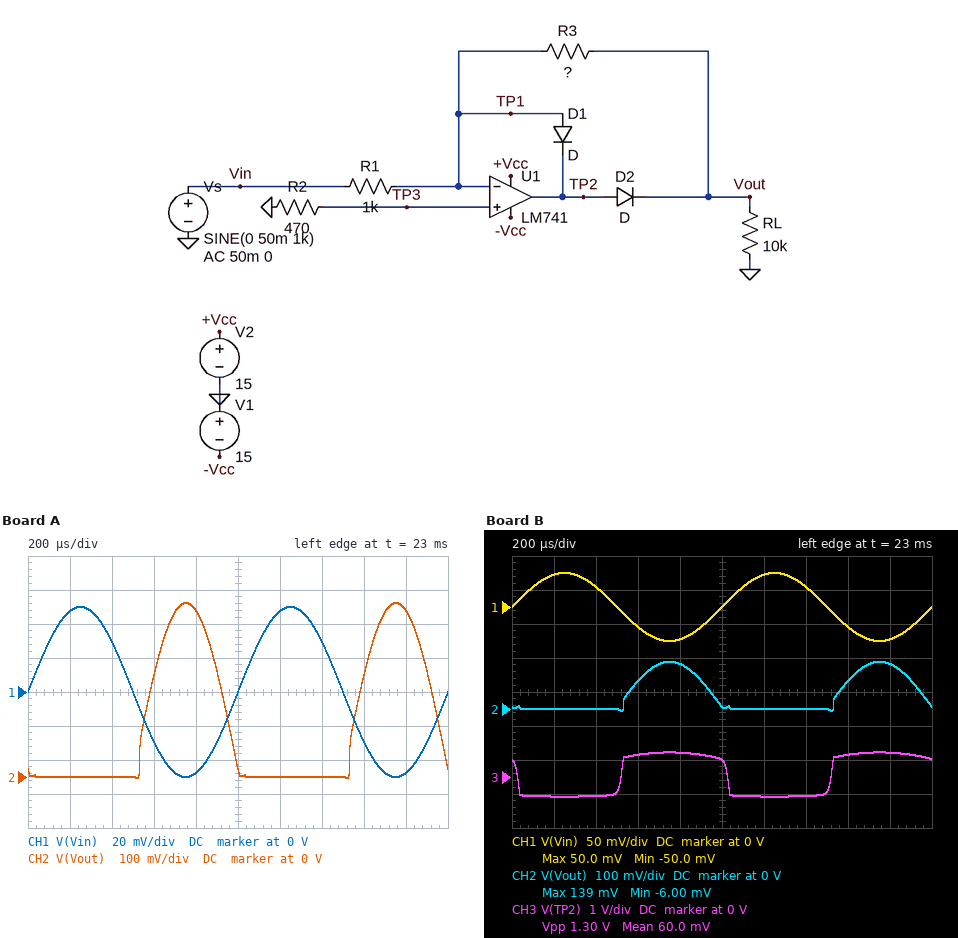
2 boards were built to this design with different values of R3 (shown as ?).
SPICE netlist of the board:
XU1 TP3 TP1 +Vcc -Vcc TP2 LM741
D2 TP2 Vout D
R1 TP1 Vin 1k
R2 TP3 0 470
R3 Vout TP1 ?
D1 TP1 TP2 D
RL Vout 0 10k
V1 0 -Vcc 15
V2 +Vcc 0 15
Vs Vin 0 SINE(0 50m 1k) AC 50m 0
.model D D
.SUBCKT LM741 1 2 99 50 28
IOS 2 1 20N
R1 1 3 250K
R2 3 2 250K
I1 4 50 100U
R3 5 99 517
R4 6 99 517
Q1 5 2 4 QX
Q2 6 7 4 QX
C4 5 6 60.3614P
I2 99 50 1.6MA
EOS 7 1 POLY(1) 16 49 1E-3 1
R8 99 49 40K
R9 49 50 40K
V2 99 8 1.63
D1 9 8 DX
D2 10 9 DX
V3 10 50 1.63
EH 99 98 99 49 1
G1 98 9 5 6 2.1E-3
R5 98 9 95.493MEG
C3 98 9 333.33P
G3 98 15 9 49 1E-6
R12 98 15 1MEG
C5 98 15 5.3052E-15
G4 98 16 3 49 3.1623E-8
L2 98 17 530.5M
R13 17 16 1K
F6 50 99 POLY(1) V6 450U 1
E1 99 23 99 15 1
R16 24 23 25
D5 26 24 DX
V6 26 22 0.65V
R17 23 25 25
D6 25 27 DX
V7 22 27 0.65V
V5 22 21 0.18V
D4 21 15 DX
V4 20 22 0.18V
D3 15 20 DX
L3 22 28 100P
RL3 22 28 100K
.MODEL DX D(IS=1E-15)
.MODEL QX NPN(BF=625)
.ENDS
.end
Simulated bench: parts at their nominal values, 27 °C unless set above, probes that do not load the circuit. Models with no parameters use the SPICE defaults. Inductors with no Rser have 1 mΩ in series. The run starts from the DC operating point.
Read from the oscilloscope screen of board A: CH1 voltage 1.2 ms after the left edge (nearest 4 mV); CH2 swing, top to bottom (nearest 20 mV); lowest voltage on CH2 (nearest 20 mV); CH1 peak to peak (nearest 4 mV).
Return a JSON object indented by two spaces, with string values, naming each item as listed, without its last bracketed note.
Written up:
{
  "CH1 voltage 1.2 ms after the left edge": "48 mV",
  "CH2 swing, top to bottom": "520 mV",
  "lowest voltage on CH2": "0 V",
  "CH1 peak to peak": "100 mV"
}
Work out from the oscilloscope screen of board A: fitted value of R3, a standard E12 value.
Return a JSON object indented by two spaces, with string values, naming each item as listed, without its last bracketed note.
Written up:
{
  "fitted value of R3, a standard E12 value": "10 kΩ"
}
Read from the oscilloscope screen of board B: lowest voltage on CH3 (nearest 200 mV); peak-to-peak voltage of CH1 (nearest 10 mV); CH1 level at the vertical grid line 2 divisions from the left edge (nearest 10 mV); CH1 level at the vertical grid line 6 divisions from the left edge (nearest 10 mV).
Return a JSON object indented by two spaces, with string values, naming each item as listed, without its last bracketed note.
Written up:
{
  "lowest voltage on CH3": "-600 mV",
  "peak-to-peak voltage of CH1": "100 mV",
  "CH1 level at the vertical grid line 2 divisions from the left edge": "30 mV",
  "CH1 level at the vertical grid line 6 divisions from the left edge": "50 mV"
}
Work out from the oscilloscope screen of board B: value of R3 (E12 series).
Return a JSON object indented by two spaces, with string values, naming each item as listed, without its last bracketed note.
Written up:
{
  "value of R3": "2.7 kΩ"
}
